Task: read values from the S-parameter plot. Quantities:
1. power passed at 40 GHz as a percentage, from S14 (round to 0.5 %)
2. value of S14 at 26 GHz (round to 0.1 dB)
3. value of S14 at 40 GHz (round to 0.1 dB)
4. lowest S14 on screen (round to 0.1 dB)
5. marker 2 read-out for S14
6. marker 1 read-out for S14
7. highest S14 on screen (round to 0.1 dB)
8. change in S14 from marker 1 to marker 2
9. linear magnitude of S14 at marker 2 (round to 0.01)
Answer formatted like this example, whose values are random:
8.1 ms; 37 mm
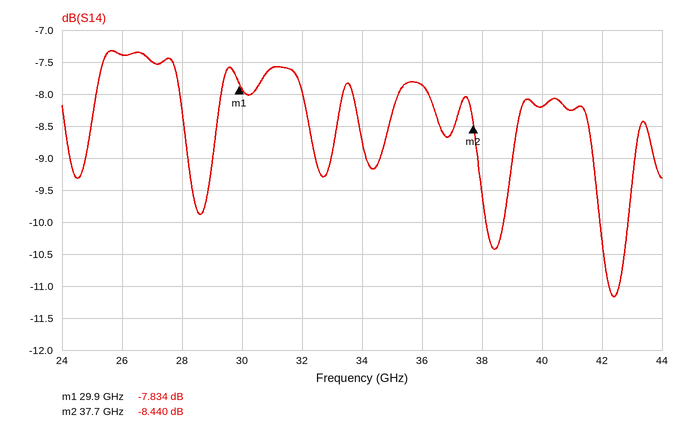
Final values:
15.0 %; -7.4 dB; -8.2 dB; -11.2 dB; -8.440 dB; -7.834 dB; -7.3 dB; -0.606 dB; 0.38
